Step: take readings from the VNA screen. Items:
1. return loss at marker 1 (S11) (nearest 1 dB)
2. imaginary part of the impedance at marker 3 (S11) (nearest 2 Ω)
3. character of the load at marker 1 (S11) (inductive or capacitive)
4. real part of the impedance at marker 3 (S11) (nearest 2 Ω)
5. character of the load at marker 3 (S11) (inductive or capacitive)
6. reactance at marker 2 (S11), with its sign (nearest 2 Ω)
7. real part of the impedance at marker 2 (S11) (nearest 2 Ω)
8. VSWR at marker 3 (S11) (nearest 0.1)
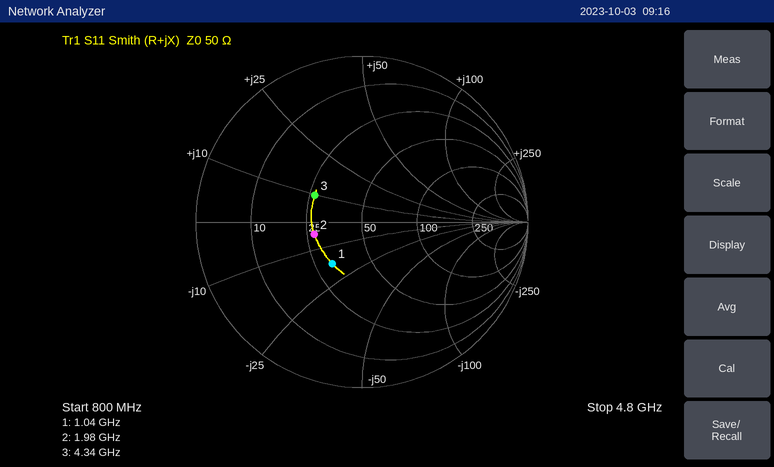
10 dB
+10 Ω
capacitive
26 Ω
inductive
-4 Ω
28 Ω
2.0
